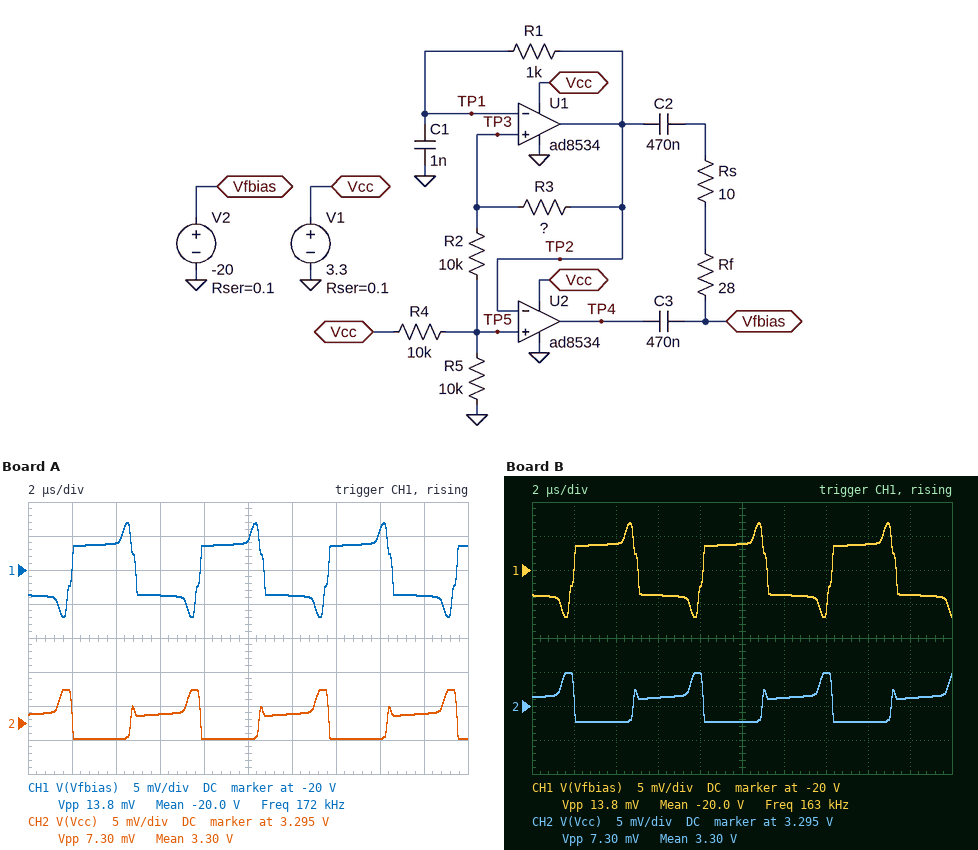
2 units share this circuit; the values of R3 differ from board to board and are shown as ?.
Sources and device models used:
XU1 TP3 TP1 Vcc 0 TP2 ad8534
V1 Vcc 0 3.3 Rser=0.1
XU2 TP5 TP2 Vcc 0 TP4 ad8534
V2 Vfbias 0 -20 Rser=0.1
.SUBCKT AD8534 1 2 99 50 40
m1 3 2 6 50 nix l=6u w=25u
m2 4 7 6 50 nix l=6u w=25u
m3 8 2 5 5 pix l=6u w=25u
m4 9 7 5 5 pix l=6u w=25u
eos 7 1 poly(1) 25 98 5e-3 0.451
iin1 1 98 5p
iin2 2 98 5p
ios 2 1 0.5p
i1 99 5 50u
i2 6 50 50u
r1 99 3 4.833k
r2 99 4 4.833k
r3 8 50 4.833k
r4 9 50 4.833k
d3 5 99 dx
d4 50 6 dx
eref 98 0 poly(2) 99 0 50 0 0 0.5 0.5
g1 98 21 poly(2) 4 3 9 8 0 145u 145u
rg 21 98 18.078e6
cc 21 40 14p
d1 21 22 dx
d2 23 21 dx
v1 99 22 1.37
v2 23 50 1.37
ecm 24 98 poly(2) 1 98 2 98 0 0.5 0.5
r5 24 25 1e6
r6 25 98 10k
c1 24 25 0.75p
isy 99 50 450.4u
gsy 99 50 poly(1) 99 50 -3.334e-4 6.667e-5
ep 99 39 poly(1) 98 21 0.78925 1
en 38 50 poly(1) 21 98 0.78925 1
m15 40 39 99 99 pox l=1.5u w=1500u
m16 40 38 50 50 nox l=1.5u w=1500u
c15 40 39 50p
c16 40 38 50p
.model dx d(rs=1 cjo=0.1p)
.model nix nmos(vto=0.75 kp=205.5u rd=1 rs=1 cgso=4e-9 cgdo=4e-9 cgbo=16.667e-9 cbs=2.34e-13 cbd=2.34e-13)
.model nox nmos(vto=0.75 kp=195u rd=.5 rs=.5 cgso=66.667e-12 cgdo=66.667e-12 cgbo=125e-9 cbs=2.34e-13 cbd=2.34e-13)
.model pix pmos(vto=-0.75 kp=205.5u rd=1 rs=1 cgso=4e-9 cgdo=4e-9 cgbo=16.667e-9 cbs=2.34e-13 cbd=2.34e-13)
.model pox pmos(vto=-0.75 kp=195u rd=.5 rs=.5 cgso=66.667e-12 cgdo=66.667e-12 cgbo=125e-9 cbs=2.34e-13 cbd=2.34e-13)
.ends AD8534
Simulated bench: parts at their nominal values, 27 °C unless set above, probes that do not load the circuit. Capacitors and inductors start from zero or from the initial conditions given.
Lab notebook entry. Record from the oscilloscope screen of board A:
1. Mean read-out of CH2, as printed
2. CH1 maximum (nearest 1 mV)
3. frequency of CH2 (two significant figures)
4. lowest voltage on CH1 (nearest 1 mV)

3.30 V
-19.993 V
170 kHz
-20.007 V
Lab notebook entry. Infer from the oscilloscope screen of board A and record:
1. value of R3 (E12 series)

3.9 kΩ
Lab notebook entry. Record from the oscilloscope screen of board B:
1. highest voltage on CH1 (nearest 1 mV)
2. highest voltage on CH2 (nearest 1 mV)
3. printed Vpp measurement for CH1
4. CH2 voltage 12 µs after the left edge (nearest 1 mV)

-19.993 V
3.300 V
13.8 mV
3.296 V
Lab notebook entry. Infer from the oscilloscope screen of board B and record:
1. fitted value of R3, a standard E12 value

3.3 kΩ
